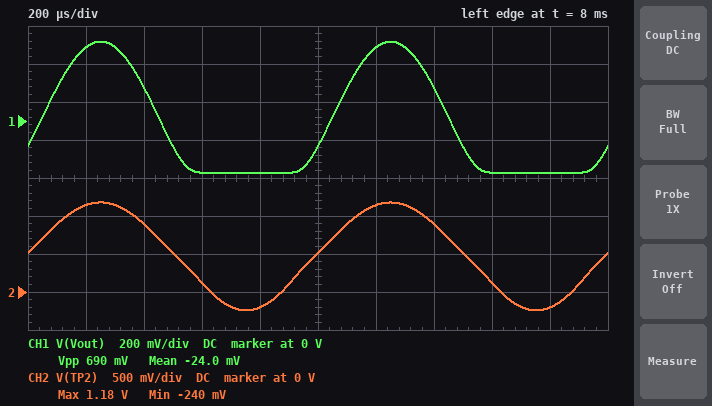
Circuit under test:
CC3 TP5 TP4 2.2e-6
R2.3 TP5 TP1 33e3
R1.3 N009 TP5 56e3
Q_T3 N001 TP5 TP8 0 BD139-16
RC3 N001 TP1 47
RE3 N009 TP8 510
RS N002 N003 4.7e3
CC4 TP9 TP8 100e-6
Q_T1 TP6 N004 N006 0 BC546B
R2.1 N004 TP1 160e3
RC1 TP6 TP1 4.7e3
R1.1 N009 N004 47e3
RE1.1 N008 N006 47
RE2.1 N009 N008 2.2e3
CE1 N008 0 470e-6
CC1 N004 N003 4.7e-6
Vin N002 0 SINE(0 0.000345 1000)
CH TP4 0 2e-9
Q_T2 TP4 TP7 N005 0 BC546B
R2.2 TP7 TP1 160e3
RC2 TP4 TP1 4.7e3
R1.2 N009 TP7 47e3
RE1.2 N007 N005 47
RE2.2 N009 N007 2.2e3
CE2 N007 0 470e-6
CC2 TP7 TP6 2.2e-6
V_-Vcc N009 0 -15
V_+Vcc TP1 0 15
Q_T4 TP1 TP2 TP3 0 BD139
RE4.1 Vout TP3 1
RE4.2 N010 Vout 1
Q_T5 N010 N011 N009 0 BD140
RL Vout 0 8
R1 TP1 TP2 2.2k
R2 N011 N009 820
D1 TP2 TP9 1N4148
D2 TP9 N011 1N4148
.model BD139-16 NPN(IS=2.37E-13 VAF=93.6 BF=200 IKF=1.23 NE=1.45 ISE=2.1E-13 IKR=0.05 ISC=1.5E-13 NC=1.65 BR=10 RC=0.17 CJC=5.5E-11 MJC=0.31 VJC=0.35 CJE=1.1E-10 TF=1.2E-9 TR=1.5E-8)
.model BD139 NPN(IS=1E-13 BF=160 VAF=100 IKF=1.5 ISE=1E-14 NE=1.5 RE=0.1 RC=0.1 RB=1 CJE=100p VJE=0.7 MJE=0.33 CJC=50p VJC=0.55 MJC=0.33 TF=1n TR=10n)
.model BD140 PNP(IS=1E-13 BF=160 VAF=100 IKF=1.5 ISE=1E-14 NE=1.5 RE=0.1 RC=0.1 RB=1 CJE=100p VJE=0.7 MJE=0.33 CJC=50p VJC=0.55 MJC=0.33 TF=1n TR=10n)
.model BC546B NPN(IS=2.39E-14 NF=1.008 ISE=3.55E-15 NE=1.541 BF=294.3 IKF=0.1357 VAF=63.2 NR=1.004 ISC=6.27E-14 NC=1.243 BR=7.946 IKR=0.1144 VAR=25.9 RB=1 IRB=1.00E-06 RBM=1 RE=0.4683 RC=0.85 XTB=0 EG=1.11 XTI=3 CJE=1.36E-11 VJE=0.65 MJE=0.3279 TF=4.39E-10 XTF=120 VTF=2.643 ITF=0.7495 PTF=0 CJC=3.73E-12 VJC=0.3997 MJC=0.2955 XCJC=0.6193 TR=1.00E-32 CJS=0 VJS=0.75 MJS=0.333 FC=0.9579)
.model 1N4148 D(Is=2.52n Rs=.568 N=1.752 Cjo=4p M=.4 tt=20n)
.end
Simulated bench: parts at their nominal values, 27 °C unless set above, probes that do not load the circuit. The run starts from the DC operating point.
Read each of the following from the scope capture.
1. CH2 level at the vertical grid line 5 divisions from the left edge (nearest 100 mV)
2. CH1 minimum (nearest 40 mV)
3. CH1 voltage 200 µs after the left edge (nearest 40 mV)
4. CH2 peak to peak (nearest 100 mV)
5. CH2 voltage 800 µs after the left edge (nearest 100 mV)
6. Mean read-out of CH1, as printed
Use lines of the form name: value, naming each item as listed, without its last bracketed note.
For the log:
CH2 level at the vertical grid line 5 divisions from the left edge: 500 mV
CH1 minimum: -280 mV
CH1 voltage 200 µs after the left edge: 400 mV
CH2 peak to peak: 1.4 V
CH2 voltage 800 µs after the left edge: -200 mV
Mean read-out of CH1, as printed: -24.0 mV
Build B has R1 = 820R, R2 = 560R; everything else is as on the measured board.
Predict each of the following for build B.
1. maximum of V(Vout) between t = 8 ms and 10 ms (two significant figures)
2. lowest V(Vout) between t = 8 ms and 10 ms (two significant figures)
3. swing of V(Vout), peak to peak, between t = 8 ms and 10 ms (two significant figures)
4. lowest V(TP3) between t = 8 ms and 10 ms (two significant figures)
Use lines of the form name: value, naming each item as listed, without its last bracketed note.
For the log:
maximum of V(Vout) between t = 8 ms and 10 ms: 910 mV
lowest V(Vout) between t = 8 ms and 10 ms: -230 mV
swing of V(Vout), peak to peak, between t = 8 ms and 10 ms: 1.1 V
lowest V(TP3) between t = 8 ms and 10 ms: -220 mV
